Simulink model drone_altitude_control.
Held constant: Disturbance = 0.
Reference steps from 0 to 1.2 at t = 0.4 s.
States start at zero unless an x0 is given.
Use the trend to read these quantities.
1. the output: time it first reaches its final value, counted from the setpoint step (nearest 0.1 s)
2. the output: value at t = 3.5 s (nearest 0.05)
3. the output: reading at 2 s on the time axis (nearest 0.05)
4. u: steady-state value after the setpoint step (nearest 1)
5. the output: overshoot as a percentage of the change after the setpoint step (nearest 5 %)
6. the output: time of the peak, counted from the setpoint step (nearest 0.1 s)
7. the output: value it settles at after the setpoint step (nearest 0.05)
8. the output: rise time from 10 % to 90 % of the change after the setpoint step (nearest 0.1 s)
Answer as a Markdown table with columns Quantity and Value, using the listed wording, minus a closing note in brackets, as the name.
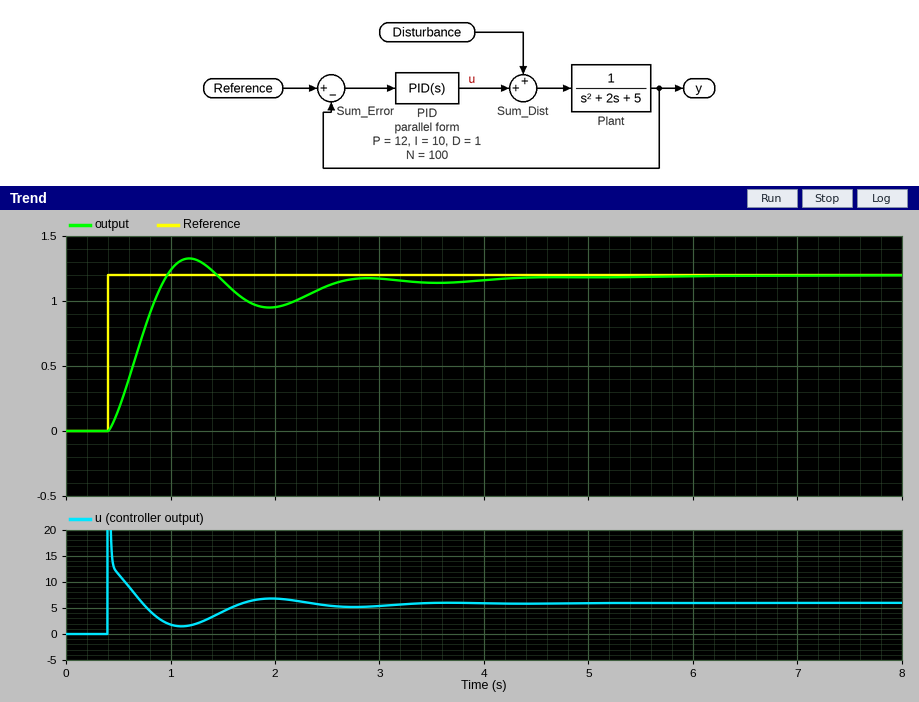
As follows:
| Quantity | Value |
|---|---|
| the output: time it first reaches its final value, counted from the setpoint step | 0.6 s |
| the output: value at t = 3.5 s | 1.15 |
| the output: reading at 2 s on the time axis | 0.95 |
| u: steady-state value after the setpoint step | 6 |
| the output: overshoot as a percentage of the change after the setpoint step | 10 % |
| the output: time of the peak, counted from the setpoint step | 0.8 s |
| the output: value it settles at after the setpoint step | 1.20 |
| the output: rise time from 10 % to 90 % of the change after the setpoint step | 0.4 s |
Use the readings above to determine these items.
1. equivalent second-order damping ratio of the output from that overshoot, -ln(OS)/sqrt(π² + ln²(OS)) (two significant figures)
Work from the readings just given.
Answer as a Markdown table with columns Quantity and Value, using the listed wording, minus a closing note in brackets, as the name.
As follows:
| Quantity | Value |
|---|---|
| equivalent second-order damping ratio of the output from that overshoot, -ln(OS)/sqrt(π² + ln²(OS)) | 0.59 |
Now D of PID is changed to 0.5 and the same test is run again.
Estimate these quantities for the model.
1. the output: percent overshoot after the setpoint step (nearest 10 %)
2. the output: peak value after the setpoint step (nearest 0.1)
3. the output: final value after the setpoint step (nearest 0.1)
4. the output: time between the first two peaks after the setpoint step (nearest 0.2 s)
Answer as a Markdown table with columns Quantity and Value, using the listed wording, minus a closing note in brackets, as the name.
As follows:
| Quantity | Value |
|---|---|
| the output: percent overshoot after the setpoint step | 20 % |
| the output: peak value after the setpoint step | 1.4 |
| the output: final value after the setpoint step | 1.2 |
| the output: time between the first two peaks after the setpoint step | 1.6 s |
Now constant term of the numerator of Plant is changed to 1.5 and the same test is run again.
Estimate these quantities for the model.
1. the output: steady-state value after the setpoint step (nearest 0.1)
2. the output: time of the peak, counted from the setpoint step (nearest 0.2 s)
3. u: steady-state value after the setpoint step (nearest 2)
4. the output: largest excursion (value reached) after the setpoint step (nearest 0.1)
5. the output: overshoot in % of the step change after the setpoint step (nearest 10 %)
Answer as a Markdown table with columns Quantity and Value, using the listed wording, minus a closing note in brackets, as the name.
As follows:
| Quantity | Value |
|---|---|
| the output: steady-state value after the setpoint step | 1.2 |
| the output: time of the peak, counted from the setpoint step | 0.6 s |
| u: steady-state value after the setpoint step | 4 |
| the output: largest excursion (value reached) after the setpoint step | 1.4 |
| the output: overshoot in % of the step change after the setpoint step | 20 % |
